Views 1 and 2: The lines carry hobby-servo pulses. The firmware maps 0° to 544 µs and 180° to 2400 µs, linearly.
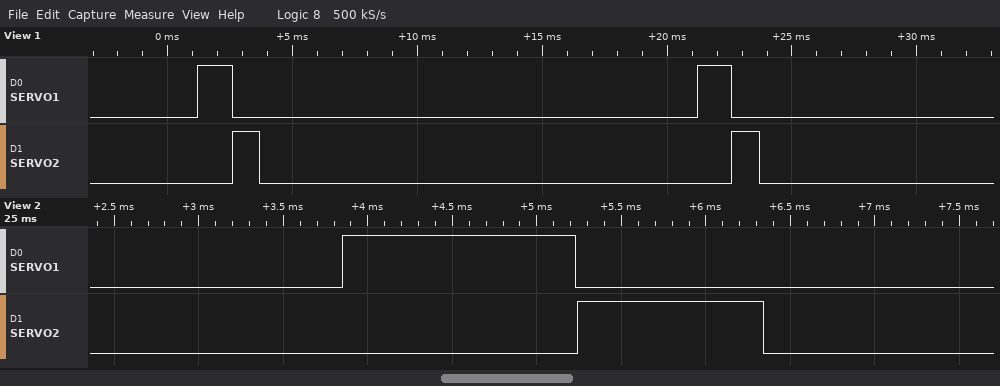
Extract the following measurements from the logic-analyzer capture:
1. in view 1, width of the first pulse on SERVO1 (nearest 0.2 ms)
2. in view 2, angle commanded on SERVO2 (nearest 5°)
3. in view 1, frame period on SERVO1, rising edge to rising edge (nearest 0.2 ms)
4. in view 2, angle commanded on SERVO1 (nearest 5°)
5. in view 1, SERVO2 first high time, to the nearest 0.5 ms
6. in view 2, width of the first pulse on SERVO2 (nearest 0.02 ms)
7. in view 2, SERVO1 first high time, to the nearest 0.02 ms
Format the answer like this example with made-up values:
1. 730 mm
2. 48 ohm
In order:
1. 1.4 ms
2. 55°
3. 20.0 ms
4. 80°
5. 1.0 ms
6. 1.10 ms
7. 1.38 ms
